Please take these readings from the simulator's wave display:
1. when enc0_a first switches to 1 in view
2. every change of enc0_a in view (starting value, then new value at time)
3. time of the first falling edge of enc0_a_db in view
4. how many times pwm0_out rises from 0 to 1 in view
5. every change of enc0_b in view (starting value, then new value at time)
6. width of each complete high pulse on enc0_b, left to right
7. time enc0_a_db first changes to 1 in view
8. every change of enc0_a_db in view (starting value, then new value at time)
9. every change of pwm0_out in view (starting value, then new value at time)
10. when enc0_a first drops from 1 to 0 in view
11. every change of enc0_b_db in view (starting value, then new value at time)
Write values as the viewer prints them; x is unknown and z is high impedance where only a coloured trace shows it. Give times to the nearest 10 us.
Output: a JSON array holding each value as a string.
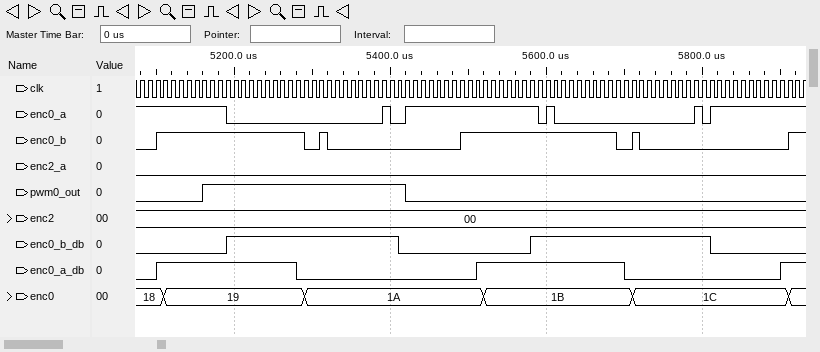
["5390 us", "1, 0 at 5190 us, 1 at 5390 us, 0 at 5400 us, 1 at 5420 us, 0 at 5590 us, 1 at 5600 us, 0 at 5610 us, 1 at 5790 us, 0 at 5800 us, 1 at 5810 us", "5280 us", "1", "0, 1 at 5100 us, 0 at 5290 us, 1 at 5310 us, 0 at 5320 us, 1 at 5490 us, 0 at 5690 us, 1 at 5710 us, 0 at 5720 us, 1 at 5910 us", "190 us, 10 us, 200 us, 10 us", "5100 us", "0, 1 at 5100 us, 0 at 5280 us, 1 at 5510 us, 0 at 5700 us, 1 at 5900 us", "0, 1 at 5160 us, 0 at 5420 us", "5190 us", "0, 1 at 5190 us, 0 at 5410 us, 1 at 5580 us, 0 at 5810 us"]
